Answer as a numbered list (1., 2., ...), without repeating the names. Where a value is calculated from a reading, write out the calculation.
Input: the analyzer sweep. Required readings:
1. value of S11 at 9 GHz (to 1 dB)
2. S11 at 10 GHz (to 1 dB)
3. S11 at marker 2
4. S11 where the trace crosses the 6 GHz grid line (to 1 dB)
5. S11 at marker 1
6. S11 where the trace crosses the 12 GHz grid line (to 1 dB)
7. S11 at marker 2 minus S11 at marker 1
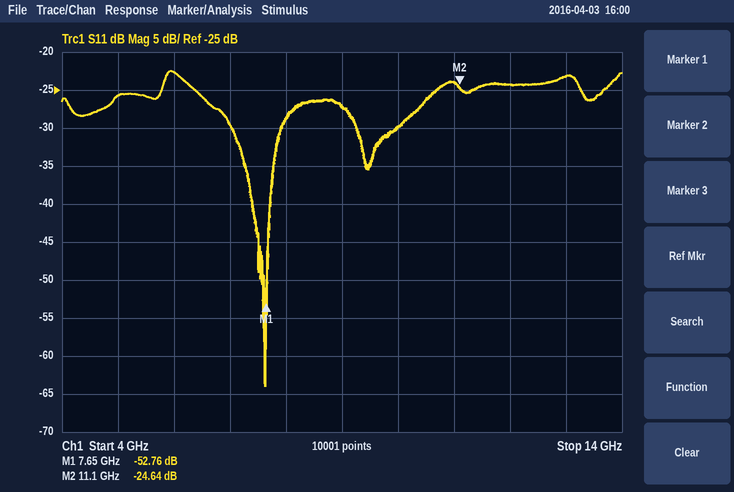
1. -27 dB
2. -30 dB
3. -24.64 dB
4. -23 dB
5. -52.76 dB
6. -24 dB
7. -24.64 − (-52.76) = 28.12 dB
